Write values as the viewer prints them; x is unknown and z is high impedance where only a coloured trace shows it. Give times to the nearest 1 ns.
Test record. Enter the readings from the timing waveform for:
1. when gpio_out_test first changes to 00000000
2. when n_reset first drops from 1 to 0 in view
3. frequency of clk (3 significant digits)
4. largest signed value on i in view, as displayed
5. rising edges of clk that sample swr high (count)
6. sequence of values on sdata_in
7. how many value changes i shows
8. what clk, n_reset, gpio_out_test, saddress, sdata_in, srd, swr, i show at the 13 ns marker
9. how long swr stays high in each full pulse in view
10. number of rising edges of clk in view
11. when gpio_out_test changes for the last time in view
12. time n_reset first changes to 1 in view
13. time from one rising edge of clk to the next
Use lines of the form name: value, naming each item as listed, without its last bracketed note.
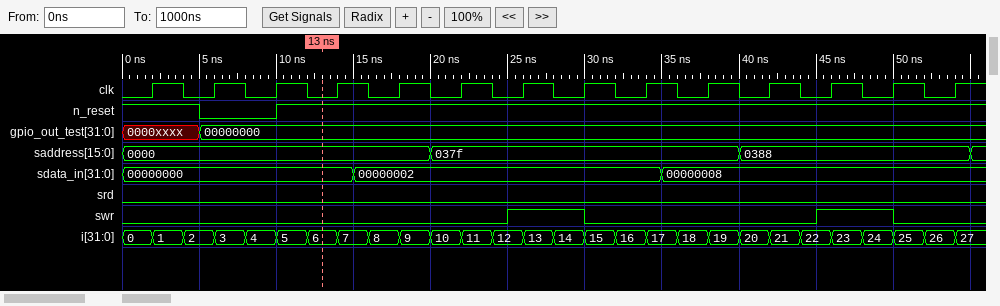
when gpio_out_test first changes to 00000000: 5 ns
when n_reset first drops from 1 to 0 in view: 5 ns
frequency of clk: 250 MHz
largest signed value on i in view, as displayed: 27
rising edges of clk that sample swr high: 4
sequence of values on sdata_in: 00000000, 00000002, 00000008
how many value changes i shows: 27
what clk, n_reset, gpio_out_test, saddress, sdata_in, srd, swr, i show at the 13 ns marker: clk=0, n_reset=1, gpio_out_test=00000000, saddress=0000, sdata_in=00000000, srd=0, swr=0, i=6
how long swr stays high in each full pulse in view: 5 ns, 5 ns
number of rising edges of clk in view: 14
when gpio_out_test changes for the last time in view: 5 ns
time n_reset first changes to 1 in view: 10 ns
time from one rising edge of clk to the next: 4 ns
